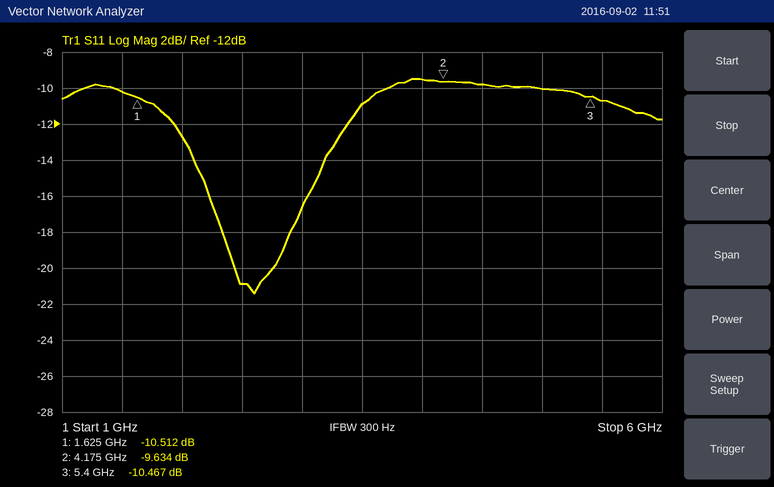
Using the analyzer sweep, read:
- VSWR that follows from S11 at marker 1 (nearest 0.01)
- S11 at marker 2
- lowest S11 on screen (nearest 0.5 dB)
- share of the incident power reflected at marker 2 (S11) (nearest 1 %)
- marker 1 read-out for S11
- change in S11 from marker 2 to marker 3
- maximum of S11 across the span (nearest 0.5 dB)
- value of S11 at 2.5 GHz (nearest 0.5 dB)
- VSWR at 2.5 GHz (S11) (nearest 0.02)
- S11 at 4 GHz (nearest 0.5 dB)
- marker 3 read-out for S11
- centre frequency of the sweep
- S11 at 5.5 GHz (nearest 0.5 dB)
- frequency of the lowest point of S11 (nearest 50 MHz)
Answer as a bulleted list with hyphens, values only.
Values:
- 1.85
- -9.634 dB
- -21.5 dB
- 11 %
- -10.512 dB
- -0.833 dB
- -9.5 dB
- -21.0 dB
- 1.20
- -9.5 dB
- -10.467 dB
- 3.5 GHz
- -10.5 dB
- 2.60 GHz
